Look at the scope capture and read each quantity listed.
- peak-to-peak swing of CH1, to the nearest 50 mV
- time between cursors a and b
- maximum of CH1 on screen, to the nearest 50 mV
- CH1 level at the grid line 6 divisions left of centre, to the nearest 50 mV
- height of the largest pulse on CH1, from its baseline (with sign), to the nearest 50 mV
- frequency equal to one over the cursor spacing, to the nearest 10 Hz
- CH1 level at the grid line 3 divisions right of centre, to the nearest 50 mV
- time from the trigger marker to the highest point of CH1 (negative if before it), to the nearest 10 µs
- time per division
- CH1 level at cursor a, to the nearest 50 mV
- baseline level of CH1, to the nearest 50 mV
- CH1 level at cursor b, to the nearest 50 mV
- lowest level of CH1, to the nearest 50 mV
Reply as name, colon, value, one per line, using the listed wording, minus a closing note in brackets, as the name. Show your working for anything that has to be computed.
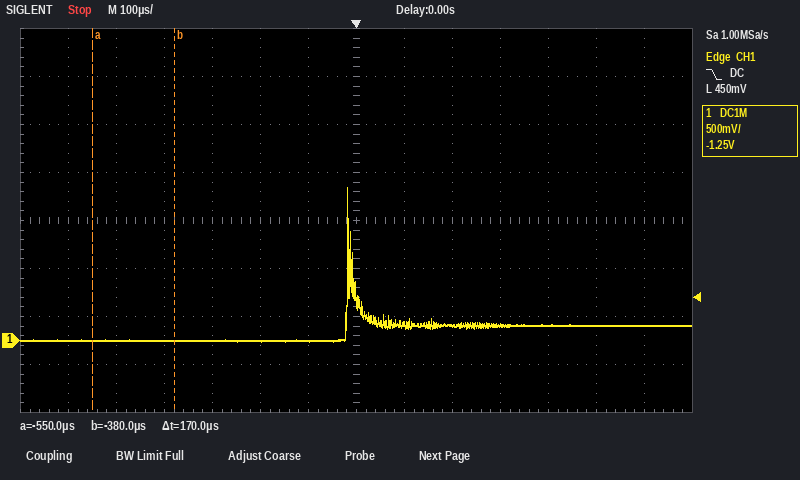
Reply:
peak-to-peak swing of CH1, to the nearest 50 mV: 1.60 V − (0 mV) = 1.60 V
time between cursors a and b: 170 µs
maximum of CH1 on screen, to the nearest 50 mV: 1.60 V
CH1 level at the grid line 6 divisions left of centre, to the nearest 50 mV: 0 mV
height of the largest pulse on CH1, from its baseline (with sign), to the nearest 50 mV: 1.60 V − (150 mV) = +1.45 V
frequency equal to one over the cursor spacing, to the nearest 10 Hz: 1 / 170 µs ≈ 5.88 kHz
CH1 level at the grid line 3 divisions right of centre, to the nearest 50 mV: 150 mV
time from the trigger marker to the highest point of CH1 (negative if before it), to the nearest 10 µs: -20 µs
time per division: 100 µs
CH1 level at cursor a, to the nearest 50 mV: 0 mV
baseline level of CH1, to the nearest 50 mV: 150 mV
CH1 level at cursor b, to the nearest 50 mV: 0 mV
lowest level of CH1, to the nearest 50 mV: 0 mV
